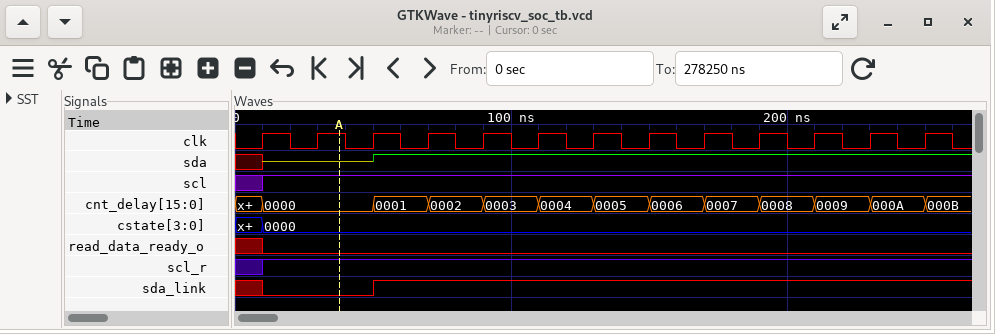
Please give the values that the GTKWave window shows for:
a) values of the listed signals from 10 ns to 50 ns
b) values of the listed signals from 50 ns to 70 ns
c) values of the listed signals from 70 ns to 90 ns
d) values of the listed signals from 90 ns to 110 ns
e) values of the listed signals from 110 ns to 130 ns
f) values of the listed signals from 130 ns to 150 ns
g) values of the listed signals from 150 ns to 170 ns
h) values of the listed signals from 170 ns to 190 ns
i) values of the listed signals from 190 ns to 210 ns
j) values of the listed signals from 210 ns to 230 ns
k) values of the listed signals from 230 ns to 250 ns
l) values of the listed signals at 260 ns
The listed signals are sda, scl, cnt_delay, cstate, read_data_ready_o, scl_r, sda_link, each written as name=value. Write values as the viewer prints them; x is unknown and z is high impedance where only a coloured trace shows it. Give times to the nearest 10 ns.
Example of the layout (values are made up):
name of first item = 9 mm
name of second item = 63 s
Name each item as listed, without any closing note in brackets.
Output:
values of the listed signals from 10 ns to 50 ns = sda=z, scl=1, cnt_delay=0000, cstate=0000, read_data_ready_o=0, scl_r=1, sda_link=0
values of the listed signals from 50 ns to 70 ns = sda=1, scl=1, cnt_delay=0001, cstate=0000, read_data_ready_o=0, scl_r=1, sda_link=1
values of the listed signals from 70 ns to 90 ns = sda=1, scl=1, cnt_delay=0002, cstate=0000, read_data_ready_o=0, scl_r=1, sda_link=1
values of the listed signals from 90 ns to 110 ns = sda=1, scl=1, cnt_delay=0003, cstate=0000, read_data_ready_o=0, scl_r=1, sda_link=1
values of the listed signals from 110 ns to 130 ns = sda=1, scl=1, cnt_delay=0004, cstate=0000, read_data_ready_o=0, scl_r=1, sda_link=1
values of the listed signals from 130 ns to 150 ns = sda=1, scl=1, cnt_delay=0005, cstate=0000, read_data_ready_o=0, scl_r=1, sda_link=1
values of the listed signals from 150 ns to 170 ns = sda=1, scl=1, cnt_delay=0006, cstate=0000, read_data_ready_o=0, scl_r=1, sda_link=1
values of the listed signals from 170 ns to 190 ns = sda=1, scl=1, cnt_delay=0007, cstate=0000, read_data_ready_o=0, scl_r=1, sda_link=1
values of the listed signals from 190 ns to 210 ns = sda=1, scl=1, cnt_delay=0008, cstate=0000, read_data_ready_o=0, scl_r=1, sda_link=1
values of the listed signals from 210 ns to 230 ns = sda=1, scl=1, cnt_delay=0009, cstate=0000, read_data_ready_o=0, scl_r=1, sda_link=1
values of the listed signals from 230 ns to 250 ns = sda=1, scl=1, cnt_delay=000A, cstate=0000, read_data_ready_o=0, scl_r=1, sda_link=1
values of the listed signals at 260 ns = sda=1, scl=1, cnt_delay=000B, cstate=0000, read_data_ready_o=0, scl_r=1, sda_link=1
